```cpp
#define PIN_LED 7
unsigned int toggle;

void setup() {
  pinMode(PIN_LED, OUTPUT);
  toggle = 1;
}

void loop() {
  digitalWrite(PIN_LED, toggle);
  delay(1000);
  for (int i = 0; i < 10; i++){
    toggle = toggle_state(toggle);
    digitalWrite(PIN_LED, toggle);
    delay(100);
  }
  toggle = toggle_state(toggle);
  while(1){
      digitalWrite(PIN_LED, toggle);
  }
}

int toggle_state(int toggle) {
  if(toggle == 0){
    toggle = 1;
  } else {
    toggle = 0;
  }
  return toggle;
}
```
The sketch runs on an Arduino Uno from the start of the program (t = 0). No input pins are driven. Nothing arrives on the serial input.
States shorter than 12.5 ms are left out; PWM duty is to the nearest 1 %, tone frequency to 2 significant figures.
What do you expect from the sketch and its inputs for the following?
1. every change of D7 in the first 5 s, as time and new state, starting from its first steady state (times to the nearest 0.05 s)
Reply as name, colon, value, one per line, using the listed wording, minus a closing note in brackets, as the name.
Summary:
every change of D7 in the first 5 s, as time and new state, starting from its first steady state: 0 s high; 1 s low; 1.1 s high; 1.2 s low; 1.3 s high; 1.4 s low; 1.5 s high; 1.6 s low; 1.7 s high; 1.8 s low; 1.9 s high; 2 s low
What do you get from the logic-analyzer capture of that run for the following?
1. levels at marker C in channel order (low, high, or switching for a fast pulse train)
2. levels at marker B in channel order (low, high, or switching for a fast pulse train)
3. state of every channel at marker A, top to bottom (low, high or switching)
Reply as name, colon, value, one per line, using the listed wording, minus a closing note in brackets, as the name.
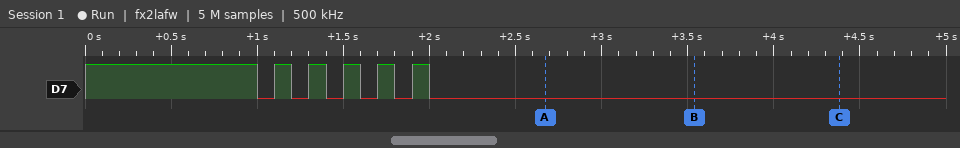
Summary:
levels at marker C in channel order: D7 low
levels at marker B in channel order: D7 low
state of every channel at marker A, top to bottom: D7 low
